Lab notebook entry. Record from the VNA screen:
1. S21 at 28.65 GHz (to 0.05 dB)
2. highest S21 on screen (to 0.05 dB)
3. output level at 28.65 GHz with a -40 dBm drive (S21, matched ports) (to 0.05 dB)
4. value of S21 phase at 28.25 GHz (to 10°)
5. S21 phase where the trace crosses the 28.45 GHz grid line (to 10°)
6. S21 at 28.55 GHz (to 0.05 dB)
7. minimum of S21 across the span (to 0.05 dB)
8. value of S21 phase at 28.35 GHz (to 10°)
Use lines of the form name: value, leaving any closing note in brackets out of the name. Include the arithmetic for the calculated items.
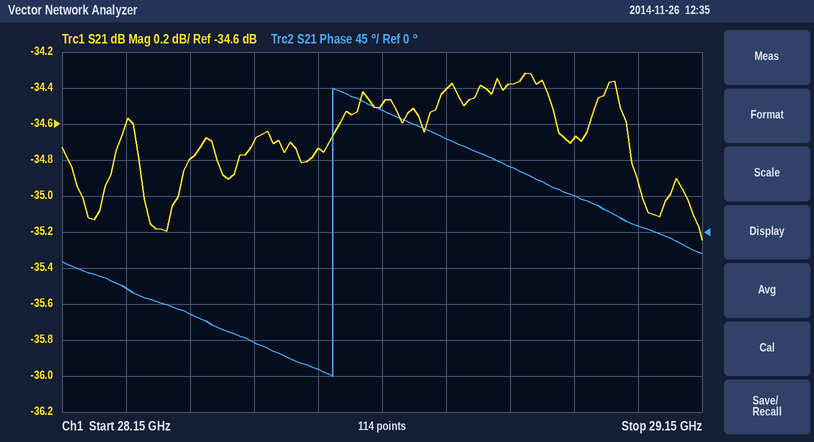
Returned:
S21 at 28.65 GHz: -34.50 dB
highest S21 on screen: -34.30 dB
output level at 28.65 GHz with a -40 dBm drive (S21, matched ports): -40 dBm + (-34.50 dB) = -74.50 dBm
value of S21 phase at 28.25 GHz: -70°
S21 phase where the trace crosses the 28.45 GHz grid line: -140°
S21 at 28.55 GHz: -34.75 dB
minimum of S21 across the span: -35.25 dB
value of S21 phase at 28.35 GHz: -100°
